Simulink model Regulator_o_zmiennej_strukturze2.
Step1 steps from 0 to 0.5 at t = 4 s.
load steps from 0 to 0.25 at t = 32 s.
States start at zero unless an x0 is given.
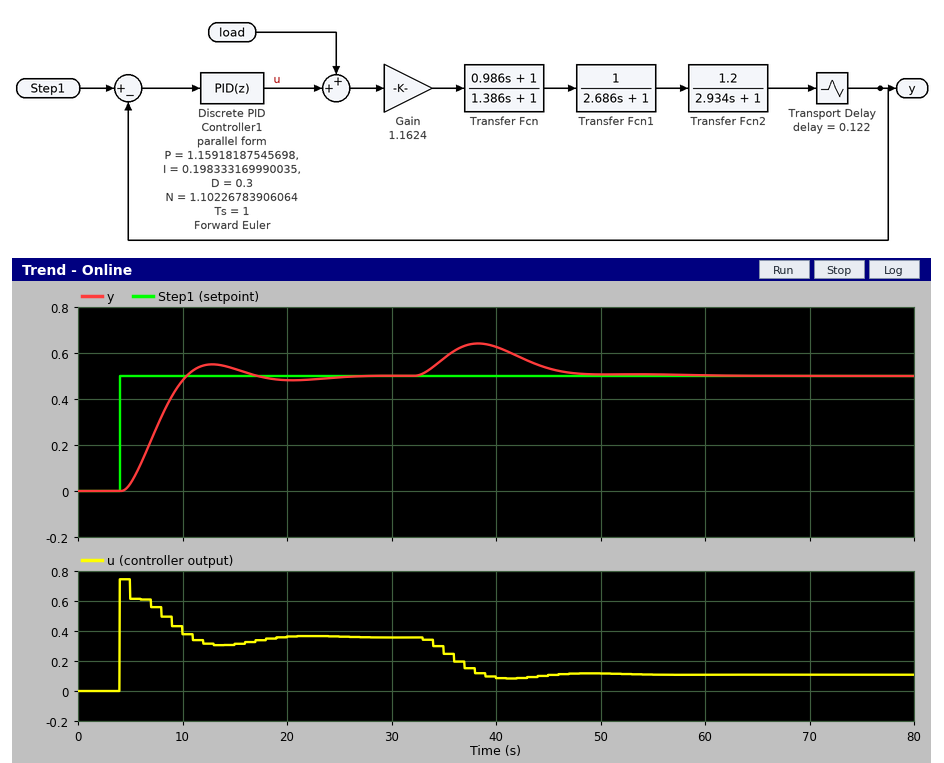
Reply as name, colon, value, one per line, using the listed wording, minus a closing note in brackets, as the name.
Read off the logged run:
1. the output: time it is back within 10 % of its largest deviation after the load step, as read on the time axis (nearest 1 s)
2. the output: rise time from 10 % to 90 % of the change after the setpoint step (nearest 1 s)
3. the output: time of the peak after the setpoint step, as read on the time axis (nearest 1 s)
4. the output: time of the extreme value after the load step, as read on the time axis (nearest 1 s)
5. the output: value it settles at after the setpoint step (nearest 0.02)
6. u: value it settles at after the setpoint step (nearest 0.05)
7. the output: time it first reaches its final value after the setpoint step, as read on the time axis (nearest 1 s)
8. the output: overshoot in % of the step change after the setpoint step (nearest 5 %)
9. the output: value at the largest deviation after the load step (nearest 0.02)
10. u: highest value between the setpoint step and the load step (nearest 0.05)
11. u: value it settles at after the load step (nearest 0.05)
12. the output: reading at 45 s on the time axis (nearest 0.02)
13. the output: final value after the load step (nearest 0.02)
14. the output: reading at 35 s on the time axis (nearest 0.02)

the output: time it is back within 10 % of its largest deviation after the load step, as read on the time axis: 47 s
the output: rise time from 10 % to 90 % of the change after the setpoint step: 4 s
the output: time of the peak after the setpoint step, as read on the time axis: 13 s
the output: time of the extreme value after the load step, as read on the time axis: 38 s
the output: value it settles at after the setpoint step: 0.50
u: value it settles at after the setpoint step: 0.35
the output: time it first reaches its final value after the setpoint step, as read on the time axis: 10 s
the output: overshoot in % of the step change after the setpoint step: 10 %
the output: value at the largest deviation after the load step: 0.64
u: highest value between the setpoint step and the load step: 0.75
u: value it settles at after the load step: 0.10
the output: reading at 45 s on the time axis: 0.54
the output: final value after the load step: 0.50
the output: reading at 35 s on the time axis: 0.58
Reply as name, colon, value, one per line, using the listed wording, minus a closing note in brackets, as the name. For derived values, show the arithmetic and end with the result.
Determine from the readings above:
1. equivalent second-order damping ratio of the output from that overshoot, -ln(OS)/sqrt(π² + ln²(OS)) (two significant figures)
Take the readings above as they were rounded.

equivalent second-order damping ratio of the output from that overshoot, -ln(OS)/sqrt(π² + ln²(OS)): ln(0.1) = -2.303; 2.303 / sqrt(9.870 + 5.302) = 0.59
